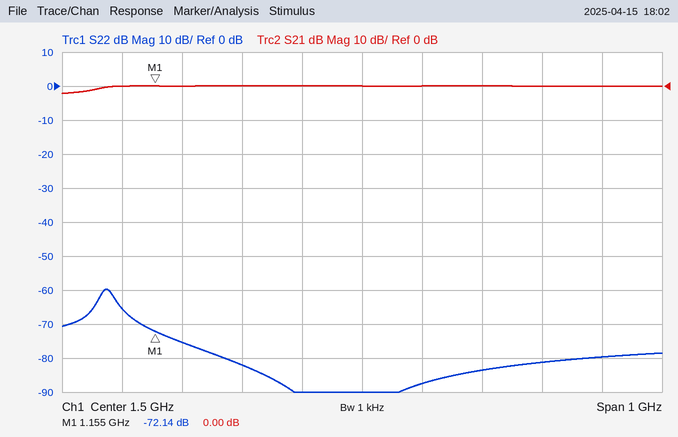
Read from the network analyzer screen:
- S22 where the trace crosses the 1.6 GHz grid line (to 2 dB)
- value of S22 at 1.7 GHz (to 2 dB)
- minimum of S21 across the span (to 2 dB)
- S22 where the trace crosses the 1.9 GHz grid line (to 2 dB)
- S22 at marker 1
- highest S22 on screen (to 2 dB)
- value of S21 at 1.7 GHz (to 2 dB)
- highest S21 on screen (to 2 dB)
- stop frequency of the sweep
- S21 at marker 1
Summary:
-88 dB
-84 dB
-2 dB
-80 dB
-72.14 dB
-60 dB
0 dB
0 dB
2 GHz
0.00 dB
